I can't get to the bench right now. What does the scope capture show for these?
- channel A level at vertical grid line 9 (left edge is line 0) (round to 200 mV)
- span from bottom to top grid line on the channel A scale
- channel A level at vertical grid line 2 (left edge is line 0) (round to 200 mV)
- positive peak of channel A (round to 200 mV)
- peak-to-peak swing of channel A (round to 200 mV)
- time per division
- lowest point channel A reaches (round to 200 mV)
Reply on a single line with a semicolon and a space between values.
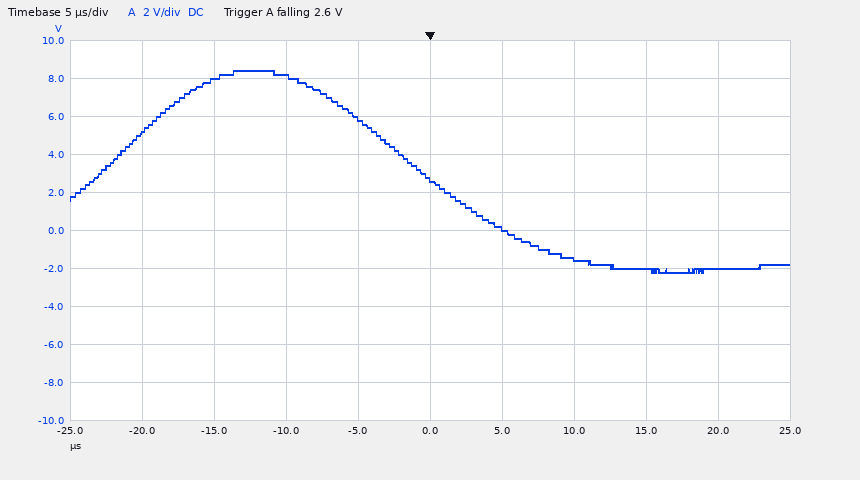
-2.0 V; 20 V; 8.0 V; 8.4 V; 10.6 V; 5 µs; -2.2 V
